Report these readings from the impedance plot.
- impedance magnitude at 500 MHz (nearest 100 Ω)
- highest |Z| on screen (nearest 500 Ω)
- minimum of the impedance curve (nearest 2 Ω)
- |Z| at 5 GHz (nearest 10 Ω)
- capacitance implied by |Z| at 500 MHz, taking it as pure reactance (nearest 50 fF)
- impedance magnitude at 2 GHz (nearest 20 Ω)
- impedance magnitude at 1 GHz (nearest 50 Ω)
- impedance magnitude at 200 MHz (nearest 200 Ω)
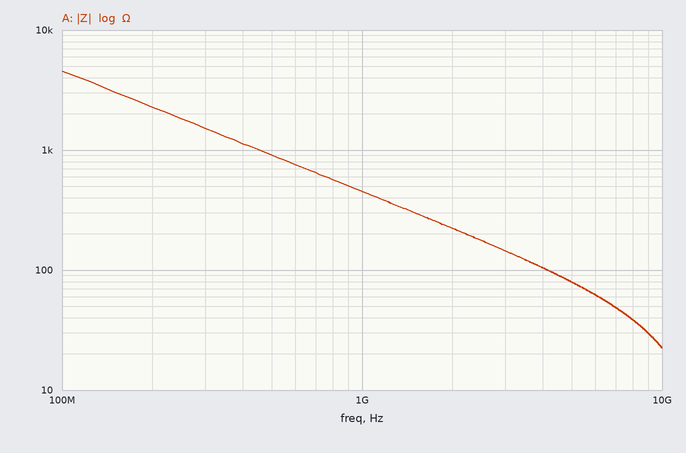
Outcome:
900 Ω
4.5 kΩ
22 Ω
80 Ω
350 fF
220 Ω
450 Ω
2.2 kΩ
